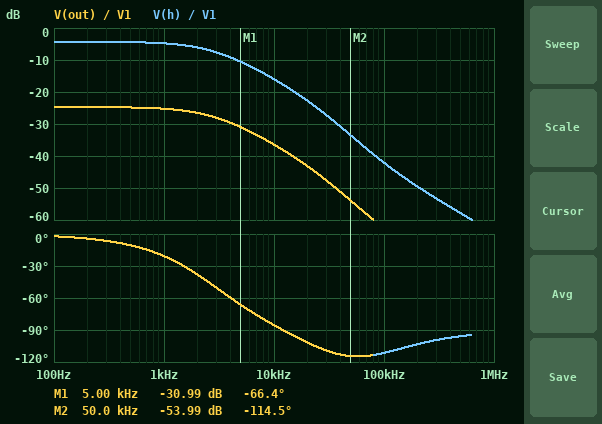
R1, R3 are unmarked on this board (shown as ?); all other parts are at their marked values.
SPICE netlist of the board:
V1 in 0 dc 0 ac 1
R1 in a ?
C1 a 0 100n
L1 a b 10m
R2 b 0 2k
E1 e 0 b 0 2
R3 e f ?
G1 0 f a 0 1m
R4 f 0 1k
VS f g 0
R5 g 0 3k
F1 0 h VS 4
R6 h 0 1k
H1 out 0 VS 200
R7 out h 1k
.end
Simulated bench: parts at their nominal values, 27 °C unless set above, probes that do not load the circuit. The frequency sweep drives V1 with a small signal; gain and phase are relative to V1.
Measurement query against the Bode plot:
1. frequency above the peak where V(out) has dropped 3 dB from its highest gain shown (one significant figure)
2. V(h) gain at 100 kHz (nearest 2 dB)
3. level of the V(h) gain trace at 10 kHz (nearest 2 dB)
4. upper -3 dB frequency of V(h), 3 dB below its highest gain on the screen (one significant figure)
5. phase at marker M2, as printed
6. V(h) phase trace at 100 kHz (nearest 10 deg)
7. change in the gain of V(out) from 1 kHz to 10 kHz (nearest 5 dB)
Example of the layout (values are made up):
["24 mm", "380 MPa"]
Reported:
["3 kHz", "-42 dB", "-16 dB", "3 kHz", "-114.5 deg", "-110 deg", "-10 dB"]
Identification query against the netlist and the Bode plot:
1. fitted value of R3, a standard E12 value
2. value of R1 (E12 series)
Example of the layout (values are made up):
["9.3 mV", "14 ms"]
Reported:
["1.2 kΩ", "820 Ω"]
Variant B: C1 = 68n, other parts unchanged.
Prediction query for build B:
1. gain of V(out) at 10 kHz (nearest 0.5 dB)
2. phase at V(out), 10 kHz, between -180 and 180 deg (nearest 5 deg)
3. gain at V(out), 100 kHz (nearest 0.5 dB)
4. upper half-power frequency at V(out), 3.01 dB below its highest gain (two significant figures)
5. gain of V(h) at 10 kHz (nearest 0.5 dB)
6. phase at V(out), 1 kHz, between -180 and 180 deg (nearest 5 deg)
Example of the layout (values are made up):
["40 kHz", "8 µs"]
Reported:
["-33.5 dB", "-80 deg", "-59.0 dB", "4.1 kHz", "-13.0 dB", "-15 deg"]
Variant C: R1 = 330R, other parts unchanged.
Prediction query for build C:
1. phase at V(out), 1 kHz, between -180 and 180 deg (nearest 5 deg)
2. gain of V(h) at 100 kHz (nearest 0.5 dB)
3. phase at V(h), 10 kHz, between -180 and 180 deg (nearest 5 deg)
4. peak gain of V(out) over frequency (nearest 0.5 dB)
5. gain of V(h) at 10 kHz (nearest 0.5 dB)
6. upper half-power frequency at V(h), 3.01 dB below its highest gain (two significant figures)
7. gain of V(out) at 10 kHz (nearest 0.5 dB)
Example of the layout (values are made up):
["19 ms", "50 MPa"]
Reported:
["-10 deg", "-34.0 dB", "-70 deg", "-23.0 dB", "-9.0 dB", "5.6 kHz", "-29.5 dB"]
